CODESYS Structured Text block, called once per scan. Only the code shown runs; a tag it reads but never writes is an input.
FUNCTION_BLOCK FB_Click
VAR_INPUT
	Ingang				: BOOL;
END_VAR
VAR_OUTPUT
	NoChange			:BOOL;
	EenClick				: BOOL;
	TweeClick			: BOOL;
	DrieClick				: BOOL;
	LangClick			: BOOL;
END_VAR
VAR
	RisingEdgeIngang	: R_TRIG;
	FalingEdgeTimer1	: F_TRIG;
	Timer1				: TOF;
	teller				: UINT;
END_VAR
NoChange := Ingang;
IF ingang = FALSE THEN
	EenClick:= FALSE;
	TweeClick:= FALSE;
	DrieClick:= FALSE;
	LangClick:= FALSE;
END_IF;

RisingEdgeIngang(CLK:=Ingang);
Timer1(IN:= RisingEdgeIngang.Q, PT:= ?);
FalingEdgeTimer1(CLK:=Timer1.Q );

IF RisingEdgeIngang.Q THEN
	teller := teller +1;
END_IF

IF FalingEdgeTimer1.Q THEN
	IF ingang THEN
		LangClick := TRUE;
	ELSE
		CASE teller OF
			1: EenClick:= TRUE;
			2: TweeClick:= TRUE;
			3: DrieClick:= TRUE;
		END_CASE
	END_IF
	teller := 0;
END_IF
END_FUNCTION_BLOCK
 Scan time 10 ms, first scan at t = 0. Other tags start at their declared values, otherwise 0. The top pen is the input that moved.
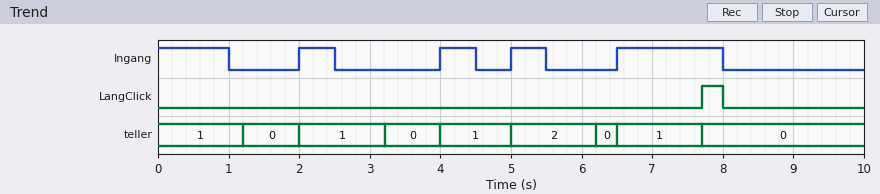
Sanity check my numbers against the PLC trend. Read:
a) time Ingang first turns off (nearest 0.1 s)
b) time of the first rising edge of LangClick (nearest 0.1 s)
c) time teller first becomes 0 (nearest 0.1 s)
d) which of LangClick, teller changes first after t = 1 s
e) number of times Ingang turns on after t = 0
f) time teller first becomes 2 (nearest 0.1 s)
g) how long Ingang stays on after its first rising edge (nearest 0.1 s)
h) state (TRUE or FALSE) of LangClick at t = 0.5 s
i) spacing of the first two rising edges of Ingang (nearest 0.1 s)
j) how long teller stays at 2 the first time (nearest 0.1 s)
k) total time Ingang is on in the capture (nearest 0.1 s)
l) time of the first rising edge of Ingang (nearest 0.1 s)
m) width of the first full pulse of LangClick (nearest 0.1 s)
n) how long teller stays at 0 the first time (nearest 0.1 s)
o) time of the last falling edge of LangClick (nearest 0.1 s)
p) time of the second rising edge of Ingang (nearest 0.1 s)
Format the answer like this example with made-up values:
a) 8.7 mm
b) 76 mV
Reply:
a) 1.0 s
b) 7.7 s
c) 1.2 s
d) teller
e) 4
f) 5.0 s
g) 0.5 s
h) FALSE
i) 2.0 s
j) 1.2 s
k) 4.0 s
l) 2.0 s
m) 0.3 s
n) 0.8 s
o) 8.0 s
p) 4.0 s
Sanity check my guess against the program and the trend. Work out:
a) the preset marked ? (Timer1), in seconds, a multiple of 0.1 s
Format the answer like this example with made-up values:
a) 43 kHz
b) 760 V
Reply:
a) 1.2 s
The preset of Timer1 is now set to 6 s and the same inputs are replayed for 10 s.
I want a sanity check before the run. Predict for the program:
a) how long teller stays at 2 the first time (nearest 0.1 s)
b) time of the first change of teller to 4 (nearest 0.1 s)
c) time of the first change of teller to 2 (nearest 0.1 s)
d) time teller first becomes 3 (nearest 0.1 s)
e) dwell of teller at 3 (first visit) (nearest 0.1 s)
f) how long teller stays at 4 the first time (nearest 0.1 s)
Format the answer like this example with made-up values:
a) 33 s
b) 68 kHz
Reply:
a) 2.0 s
b) 5.0 s
c) 2.0 s
d) 4.0 s
e) 1.0 s
f) 1.5 s
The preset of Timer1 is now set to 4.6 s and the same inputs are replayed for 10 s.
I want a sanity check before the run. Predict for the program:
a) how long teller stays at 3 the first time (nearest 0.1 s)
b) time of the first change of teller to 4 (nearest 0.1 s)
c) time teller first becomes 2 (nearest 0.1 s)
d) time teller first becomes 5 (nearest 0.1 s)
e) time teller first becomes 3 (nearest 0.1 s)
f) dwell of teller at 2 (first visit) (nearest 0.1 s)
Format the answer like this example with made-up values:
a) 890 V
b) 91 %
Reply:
a) 1.0 s
b) 5.0 s
c) 2.0 s
d) 6.5 s
e) 4.0 s
f) 2.0 s
